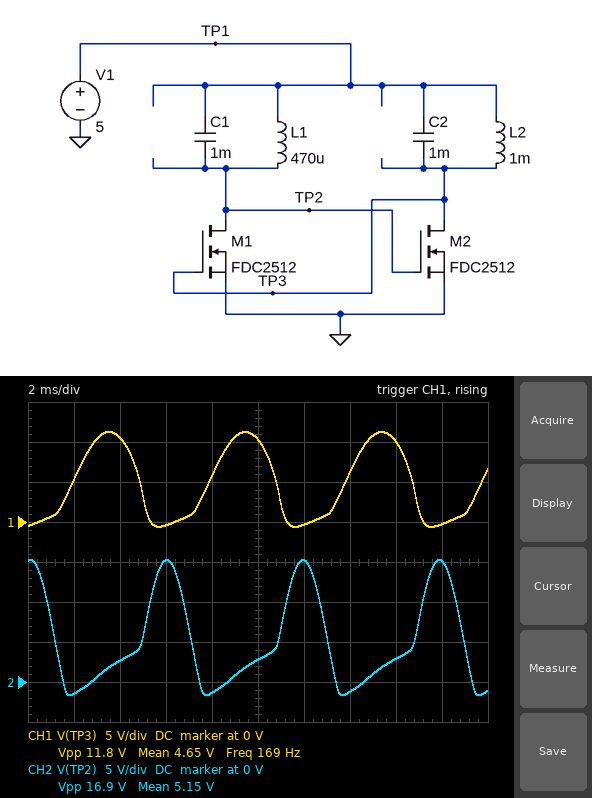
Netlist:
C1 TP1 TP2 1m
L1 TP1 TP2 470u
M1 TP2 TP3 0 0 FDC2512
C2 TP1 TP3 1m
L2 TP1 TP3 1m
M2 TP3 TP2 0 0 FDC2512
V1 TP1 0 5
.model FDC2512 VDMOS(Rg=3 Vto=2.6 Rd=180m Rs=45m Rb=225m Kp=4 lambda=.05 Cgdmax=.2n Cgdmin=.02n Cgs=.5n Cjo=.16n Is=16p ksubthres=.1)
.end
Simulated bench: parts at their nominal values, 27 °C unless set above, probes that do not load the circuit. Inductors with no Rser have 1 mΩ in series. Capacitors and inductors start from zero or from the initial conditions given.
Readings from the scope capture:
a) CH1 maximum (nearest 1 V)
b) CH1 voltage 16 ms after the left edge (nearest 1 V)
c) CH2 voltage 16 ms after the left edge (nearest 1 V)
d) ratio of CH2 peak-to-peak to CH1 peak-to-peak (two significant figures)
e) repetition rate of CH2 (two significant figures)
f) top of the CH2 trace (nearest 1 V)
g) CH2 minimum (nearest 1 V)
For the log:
11 V
10 V
3 V
1.4
170 Hz
15 V
-2 V
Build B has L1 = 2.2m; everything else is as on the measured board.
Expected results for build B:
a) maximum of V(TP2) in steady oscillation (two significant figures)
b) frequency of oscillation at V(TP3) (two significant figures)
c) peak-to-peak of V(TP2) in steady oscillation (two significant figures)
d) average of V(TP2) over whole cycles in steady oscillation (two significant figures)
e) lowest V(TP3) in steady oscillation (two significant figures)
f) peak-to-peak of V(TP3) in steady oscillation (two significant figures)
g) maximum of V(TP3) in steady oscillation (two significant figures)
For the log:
11 V
110 Hz
12 V
5.0 V
-1.8 V
19 V
17 V
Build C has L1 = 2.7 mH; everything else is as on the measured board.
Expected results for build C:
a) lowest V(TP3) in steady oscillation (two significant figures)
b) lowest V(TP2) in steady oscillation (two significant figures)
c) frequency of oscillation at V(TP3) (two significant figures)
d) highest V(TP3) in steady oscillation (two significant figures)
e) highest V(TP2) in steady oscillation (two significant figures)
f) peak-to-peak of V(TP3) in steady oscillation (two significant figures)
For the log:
-2.1 V
-490 mV
100 Hz
18 V
11 V
20 V
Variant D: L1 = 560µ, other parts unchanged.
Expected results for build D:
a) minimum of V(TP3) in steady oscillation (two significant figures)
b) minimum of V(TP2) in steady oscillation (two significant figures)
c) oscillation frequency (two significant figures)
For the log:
-710 mV
-1.5 V
160 Hz
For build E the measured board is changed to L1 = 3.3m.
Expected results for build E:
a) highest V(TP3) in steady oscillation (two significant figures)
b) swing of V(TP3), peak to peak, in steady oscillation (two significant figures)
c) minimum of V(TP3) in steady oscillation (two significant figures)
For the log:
19 V
21 V
-2.3 V
